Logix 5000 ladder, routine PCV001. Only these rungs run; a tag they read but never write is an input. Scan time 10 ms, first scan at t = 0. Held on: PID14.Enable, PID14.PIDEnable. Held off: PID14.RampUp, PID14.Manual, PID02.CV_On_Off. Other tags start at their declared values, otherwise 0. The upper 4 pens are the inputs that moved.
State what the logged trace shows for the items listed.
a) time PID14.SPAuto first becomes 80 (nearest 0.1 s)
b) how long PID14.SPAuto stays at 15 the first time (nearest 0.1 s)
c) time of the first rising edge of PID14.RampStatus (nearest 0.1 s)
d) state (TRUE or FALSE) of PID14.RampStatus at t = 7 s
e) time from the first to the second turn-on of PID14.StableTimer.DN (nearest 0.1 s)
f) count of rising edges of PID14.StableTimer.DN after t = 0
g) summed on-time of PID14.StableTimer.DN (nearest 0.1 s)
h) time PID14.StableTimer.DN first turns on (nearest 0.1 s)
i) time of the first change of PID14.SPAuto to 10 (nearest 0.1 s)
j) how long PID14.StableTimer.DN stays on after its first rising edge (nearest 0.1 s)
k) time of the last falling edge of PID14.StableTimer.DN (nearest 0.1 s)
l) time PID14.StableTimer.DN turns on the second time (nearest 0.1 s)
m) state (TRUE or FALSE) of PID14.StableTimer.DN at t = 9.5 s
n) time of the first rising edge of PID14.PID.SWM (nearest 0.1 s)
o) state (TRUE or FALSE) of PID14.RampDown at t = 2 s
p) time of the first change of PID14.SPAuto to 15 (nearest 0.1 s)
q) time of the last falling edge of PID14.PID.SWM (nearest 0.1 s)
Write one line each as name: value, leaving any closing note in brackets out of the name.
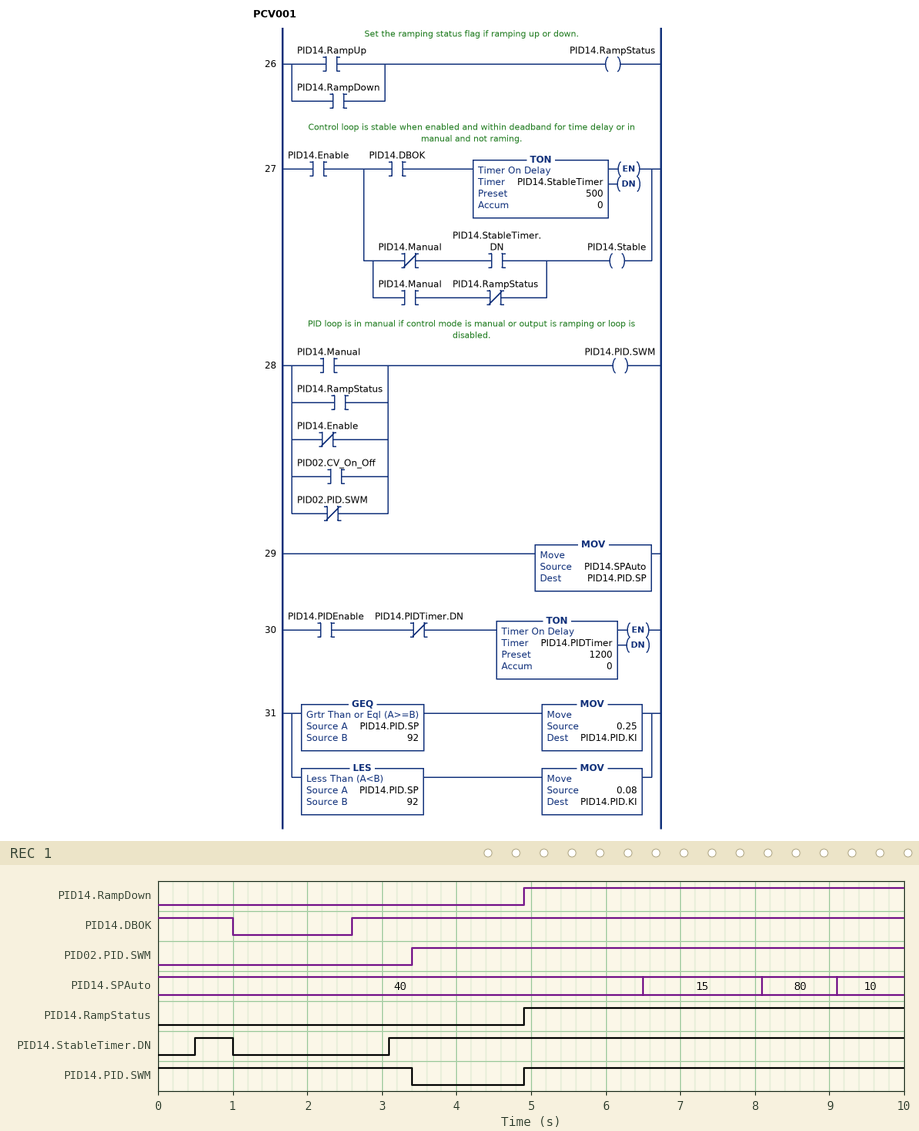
time PID14.SPAuto first becomes 80: 8.1 s
how long PID14.SPAuto stays at 15 the first time: 1.6 s
time of the first rising edge of PID14.RampStatus: 4.9 s
state (TRUE or FALSE) of PID14.RampStatus at t = 7 s: TRUE
time from the first to the second turn-on of PID14.StableTimer.DN: 2.6 s
count of rising edges of PID14.StableTimer.DN after t = 0: 2
summed on-time of PID14.StableTimer.DN: 7.4 s
time PID14.StableTimer.DN first turns on: 0.5 s
time of the first change of PID14.SPAuto to 10: 9.1 s
how long PID14.StableTimer.DN stays on after its first rising edge: 0.5 s
time of the last falling edge of PID14.StableTimer.DN: 1.0 s
time PID14.StableTimer.DN turns on the second time: 3.1 s
state (TRUE or FALSE) of PID14.StableTimer.DN at t = 9.5 s: TRUE
time of the first rising edge of PID14.PID.SWM: 4.9 s
state (TRUE or FALSE) of PID14.RampDown at t = 2 s: FALSE
time of the first change of PID14.SPAuto to 15: 6.5 s
time of the last falling edge of PID14.PID.SWM: 3.4 s
